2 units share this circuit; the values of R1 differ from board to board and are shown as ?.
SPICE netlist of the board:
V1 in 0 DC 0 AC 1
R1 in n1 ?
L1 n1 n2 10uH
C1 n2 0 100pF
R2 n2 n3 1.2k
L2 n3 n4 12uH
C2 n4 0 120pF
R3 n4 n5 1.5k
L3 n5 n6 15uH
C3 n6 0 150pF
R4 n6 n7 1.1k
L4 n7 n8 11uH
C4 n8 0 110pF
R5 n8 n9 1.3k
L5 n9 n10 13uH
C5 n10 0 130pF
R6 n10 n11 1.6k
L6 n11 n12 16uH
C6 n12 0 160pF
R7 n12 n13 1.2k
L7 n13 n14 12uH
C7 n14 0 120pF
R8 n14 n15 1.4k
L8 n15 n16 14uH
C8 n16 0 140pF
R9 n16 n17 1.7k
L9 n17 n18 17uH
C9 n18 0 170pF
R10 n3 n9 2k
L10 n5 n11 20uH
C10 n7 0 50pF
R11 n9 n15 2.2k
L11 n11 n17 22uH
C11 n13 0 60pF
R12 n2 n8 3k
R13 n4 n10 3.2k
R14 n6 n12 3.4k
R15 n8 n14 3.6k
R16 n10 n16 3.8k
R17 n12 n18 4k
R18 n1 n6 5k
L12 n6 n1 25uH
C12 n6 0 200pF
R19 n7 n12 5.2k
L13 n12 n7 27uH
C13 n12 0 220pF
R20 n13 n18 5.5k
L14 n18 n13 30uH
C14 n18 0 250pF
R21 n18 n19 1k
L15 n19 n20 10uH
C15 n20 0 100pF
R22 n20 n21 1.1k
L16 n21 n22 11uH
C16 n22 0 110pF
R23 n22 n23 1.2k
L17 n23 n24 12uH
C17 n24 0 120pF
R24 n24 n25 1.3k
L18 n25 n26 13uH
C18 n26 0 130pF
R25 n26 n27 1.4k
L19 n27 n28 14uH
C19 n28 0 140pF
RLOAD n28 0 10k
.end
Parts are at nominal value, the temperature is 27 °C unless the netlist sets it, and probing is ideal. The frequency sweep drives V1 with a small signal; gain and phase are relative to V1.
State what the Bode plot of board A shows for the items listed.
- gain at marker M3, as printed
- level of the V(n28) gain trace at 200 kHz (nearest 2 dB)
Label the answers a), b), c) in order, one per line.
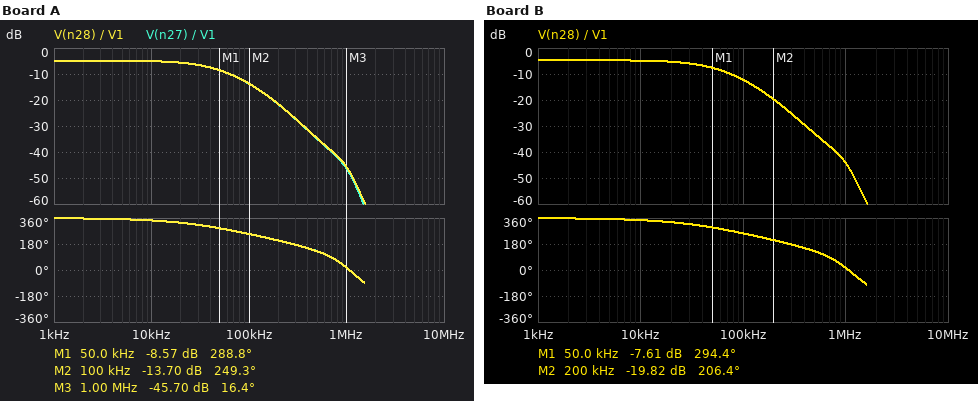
a) -45.70 dB
b) -22 dB
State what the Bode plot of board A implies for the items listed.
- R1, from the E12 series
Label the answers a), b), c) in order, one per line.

a) 1.5 kΩ
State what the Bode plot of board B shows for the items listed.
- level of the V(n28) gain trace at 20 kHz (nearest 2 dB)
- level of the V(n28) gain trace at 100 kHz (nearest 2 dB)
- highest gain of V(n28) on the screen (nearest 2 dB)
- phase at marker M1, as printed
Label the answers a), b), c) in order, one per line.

a) -6 dB
b) -12 dB
c) -4 dB
d) 294.4 deg
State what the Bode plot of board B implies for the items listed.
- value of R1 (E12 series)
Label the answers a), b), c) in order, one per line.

a) 1.2 kΩ
